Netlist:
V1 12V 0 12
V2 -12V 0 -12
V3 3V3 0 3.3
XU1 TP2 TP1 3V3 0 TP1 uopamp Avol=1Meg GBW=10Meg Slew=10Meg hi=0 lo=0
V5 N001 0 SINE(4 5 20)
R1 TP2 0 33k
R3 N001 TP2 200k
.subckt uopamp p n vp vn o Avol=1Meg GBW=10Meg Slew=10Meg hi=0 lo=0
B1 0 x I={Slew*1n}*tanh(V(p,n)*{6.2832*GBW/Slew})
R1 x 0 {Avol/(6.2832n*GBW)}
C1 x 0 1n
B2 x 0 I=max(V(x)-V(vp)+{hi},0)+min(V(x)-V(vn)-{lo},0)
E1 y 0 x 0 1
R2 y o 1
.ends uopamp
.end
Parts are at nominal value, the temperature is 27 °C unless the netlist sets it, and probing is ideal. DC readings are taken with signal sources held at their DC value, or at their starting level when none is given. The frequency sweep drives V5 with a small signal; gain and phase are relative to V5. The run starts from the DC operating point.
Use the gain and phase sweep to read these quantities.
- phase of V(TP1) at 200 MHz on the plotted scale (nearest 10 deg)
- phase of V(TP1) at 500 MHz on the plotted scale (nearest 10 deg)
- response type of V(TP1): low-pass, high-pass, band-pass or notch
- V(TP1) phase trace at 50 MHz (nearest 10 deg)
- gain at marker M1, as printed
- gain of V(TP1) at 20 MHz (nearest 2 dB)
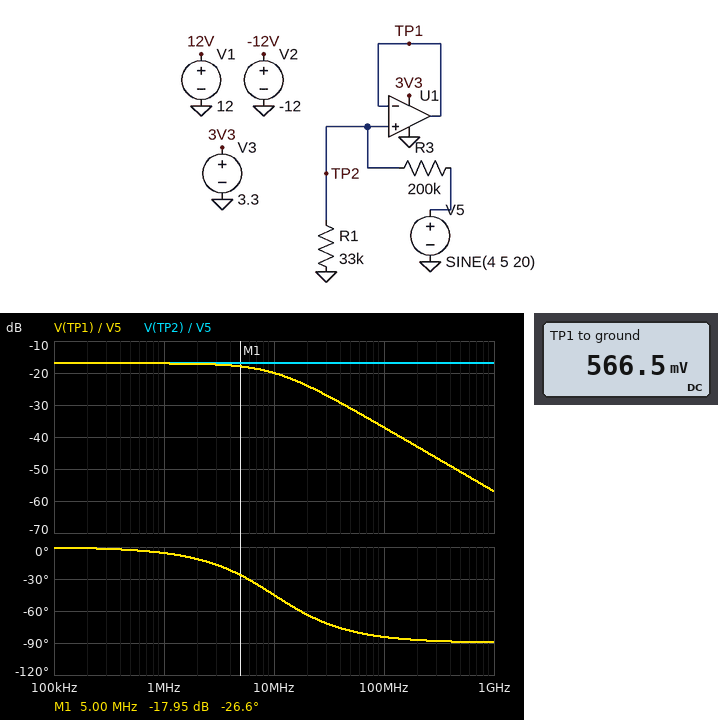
-90 deg
-90 deg
low-pass
-80 deg
-17.95 dB
-24 dB
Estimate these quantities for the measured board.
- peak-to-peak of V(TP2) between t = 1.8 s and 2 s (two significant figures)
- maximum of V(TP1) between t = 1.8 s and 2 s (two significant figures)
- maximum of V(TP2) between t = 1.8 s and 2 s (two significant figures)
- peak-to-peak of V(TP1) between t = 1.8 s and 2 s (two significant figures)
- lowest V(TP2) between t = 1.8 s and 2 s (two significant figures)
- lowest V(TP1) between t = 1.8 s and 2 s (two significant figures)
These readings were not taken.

1.4 V
1.3 V
1.3 V
1.3 V
-140 mV
-6.9 mV
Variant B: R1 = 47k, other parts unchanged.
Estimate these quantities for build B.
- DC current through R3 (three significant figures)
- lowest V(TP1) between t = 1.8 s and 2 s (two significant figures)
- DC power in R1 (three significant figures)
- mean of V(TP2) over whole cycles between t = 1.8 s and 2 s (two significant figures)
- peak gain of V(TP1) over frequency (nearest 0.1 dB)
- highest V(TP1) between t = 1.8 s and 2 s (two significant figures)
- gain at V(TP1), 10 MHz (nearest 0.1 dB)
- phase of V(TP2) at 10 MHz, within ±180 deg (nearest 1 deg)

16.2 µA
-8.2 mV
12.3 µW
760 mV
-14.4 dB
1.7 V
-17.4 dB
0 deg
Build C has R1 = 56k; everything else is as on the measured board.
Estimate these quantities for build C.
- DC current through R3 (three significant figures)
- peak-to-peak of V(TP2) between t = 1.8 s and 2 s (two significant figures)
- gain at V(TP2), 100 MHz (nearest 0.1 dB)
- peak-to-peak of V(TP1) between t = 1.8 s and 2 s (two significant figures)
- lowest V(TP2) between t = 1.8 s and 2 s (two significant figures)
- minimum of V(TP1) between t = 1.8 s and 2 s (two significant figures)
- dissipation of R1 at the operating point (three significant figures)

15.6 µA
2.2 V
-13.2 dB
2.0 V
-220 mV
-8.7 mV
13.7 µW
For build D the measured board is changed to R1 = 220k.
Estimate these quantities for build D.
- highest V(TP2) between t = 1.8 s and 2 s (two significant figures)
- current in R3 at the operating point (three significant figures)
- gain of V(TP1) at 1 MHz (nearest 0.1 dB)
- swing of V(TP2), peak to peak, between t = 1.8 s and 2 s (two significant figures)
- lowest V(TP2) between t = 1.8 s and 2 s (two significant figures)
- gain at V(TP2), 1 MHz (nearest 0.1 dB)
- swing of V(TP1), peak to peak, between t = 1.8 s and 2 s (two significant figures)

4.7 V
9.52 µA
-5.7 dB
5.2 V
-520 mV
-5.6 dB
3.3 V
